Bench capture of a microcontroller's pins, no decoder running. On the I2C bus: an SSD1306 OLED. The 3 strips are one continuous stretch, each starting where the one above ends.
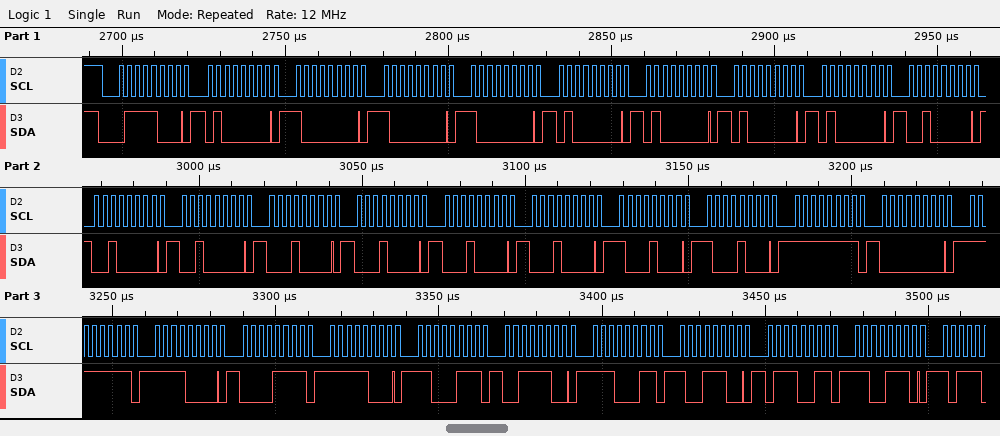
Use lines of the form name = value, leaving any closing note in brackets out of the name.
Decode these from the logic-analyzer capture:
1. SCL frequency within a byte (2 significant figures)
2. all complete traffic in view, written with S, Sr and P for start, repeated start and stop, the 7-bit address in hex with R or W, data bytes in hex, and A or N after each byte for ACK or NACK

SCL frequency within a byte = 400 kHz
all complete traffic in view, written with S, Sr and P for start, repeated start and stop, the 7-bit address in hex with R or W, data bytes in hex, and A or N after each byte for ACK or NACK = S 3CW A 40 A 80 A 80 A 80 A 40 A 40 A 40 A 40 A 20 A 20 A 20 A 10 A 10 A 10 A 10 A 88 A 88 A FF A 00 A FF A F0 A 0F A F8 A C7 A 3C A E3 A 9C A 73 A CE A
